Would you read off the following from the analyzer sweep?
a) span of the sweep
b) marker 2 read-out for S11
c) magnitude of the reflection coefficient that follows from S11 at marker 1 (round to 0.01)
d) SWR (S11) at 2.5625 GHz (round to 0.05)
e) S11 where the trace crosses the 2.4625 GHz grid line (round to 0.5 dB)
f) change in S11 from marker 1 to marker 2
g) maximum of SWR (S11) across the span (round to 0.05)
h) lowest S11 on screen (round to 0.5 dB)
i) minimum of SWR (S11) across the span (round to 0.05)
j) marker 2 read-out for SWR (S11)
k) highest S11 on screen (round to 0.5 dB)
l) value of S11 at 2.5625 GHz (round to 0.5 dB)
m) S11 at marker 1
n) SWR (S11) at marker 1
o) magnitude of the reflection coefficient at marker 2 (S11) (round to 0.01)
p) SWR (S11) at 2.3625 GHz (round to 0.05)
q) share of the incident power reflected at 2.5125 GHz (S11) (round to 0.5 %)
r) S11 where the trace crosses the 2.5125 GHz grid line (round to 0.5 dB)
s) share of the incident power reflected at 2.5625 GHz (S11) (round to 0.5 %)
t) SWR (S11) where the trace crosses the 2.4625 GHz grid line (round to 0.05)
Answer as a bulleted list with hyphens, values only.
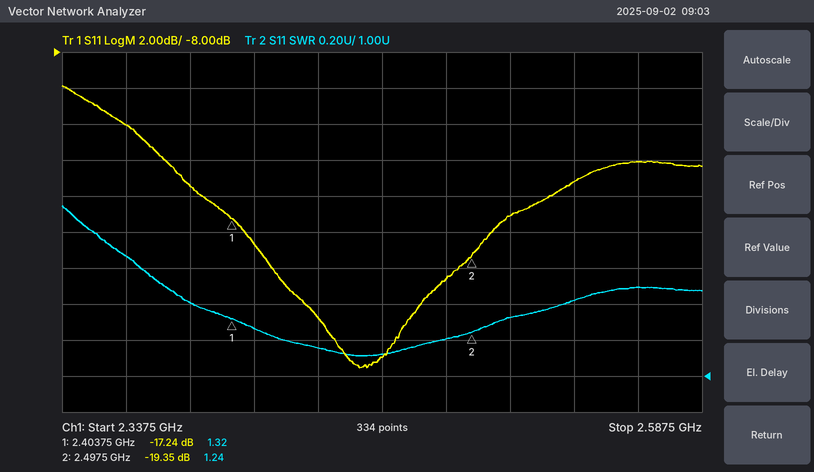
- 250 MHz
- -19.35 dB
- 0.14
- 1.50
- -25.0 dB
- -2.11 dB
- 1.95
- -25.5 dB
- 1.10
- 1.24
- -10.0 dB
- -14.0 dB
- -17.24 dB
- 1.32
- 0.11
- 1.65
- 2.0 %
- -17.0 dB
- 4.0 %
- 1.10
